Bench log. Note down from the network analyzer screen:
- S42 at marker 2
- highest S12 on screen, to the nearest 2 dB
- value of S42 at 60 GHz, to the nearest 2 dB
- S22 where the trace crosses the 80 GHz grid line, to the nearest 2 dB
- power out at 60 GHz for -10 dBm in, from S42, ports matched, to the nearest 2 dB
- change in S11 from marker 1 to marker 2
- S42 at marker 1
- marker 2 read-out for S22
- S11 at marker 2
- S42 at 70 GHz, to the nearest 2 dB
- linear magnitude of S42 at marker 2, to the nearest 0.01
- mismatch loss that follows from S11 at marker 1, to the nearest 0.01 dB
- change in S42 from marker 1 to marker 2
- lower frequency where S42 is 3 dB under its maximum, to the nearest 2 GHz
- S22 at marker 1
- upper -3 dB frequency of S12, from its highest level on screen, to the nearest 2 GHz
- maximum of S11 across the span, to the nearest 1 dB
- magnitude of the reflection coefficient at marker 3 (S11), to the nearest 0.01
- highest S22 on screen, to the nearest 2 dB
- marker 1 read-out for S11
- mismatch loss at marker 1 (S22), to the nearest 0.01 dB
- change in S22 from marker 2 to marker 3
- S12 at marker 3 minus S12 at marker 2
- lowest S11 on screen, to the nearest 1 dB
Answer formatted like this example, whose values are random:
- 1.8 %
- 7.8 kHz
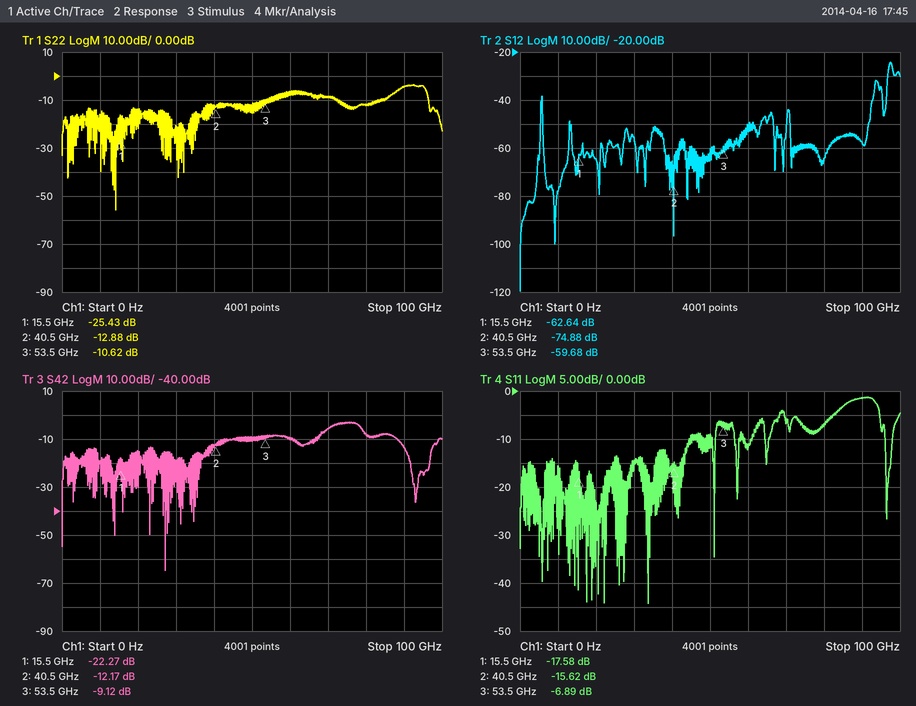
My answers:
- -12.17 dB
- -24 dB
- -10 dB
- -12 dB
- -20 dBm
- 1.96 dB
- -22.27 dB
- -12.88 dB
- -15.62 dB
- -6 dB
- 0.25
- 0.08 dB
- 10.10 dB
- 70 GHz
- -25.43 dB
- 98 GHz
- -1 dB
- 0.45
- -4 dB
- -17.58 dB
- 0.01 dB
- 2.26 dB
- 15.20 dB
- -44 dB
